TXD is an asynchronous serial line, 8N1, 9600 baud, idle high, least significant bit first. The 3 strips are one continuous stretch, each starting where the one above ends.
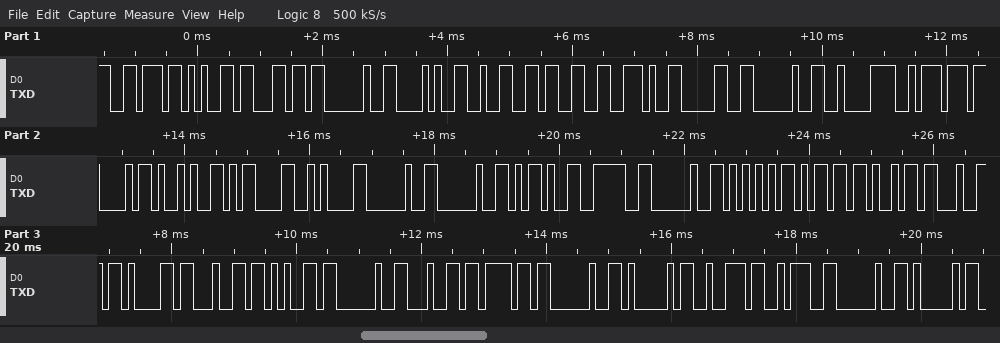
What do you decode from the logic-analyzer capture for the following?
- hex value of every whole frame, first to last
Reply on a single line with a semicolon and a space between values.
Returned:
76 65 6C 20 28 32 33 2E 30 20 C2 BA 43 29 0D 0A 20 20 2D 3E 20 55 6D 69 64 61 64 65 20 64 6F 20 41 72 3A 20 41
